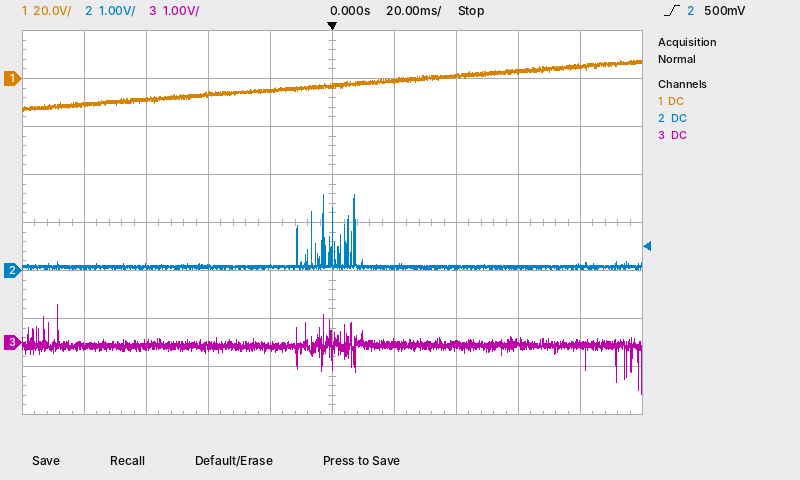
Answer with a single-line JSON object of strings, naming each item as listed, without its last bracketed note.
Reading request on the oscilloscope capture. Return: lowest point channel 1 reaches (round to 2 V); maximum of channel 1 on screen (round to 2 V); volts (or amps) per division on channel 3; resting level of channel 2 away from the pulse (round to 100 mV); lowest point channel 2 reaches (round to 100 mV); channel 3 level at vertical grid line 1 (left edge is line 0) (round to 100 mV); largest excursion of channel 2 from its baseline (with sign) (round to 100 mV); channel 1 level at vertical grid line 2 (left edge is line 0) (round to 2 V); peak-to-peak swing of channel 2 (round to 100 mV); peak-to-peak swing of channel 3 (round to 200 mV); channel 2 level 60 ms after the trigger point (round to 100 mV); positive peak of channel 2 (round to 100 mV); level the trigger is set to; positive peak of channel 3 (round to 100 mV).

{"lowest point channel 1 reaches": "-14 V", "maximum of channel 1 on screen": "8 V", "volts (or amps) per division on channel 3": "1 V", "resting level of channel 2 away from the pulse": "100 mV", "lowest point channel 2 reaches": "0.0 V", "channel 3 level at vertical grid line 1 (left edge is line 0)": "-100 mV", "largest excursion of channel 2 from its baseline (with sign)": "+1.5 V", "channel 1 level at vertical grid line 2 (left edge is line 0)": "-8 V", "peak-to-peak swing of channel 2": "1.6 V", "peak-to-peak swing of channel 3": "1.8 V", "channel 2 level 60 ms after the trigger point": "100 mV", "positive peak of channel 2": "1.6 V", "level the trigger is set to": "500 mV", "positive peak of channel 3": "800 mV"}
